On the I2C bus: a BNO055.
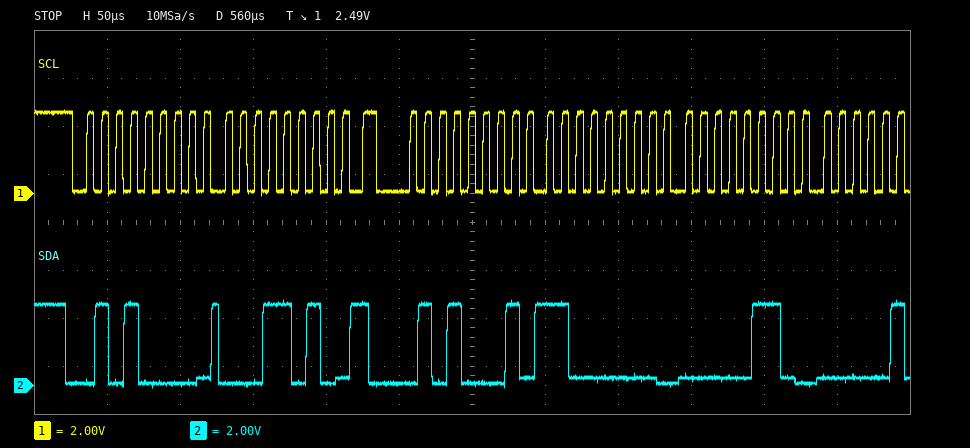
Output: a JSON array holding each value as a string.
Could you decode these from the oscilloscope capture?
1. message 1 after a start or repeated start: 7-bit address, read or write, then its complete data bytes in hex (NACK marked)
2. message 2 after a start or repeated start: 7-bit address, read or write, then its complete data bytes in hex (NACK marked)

["0x28 write: 1A", "0x28 read: C0 06"]
